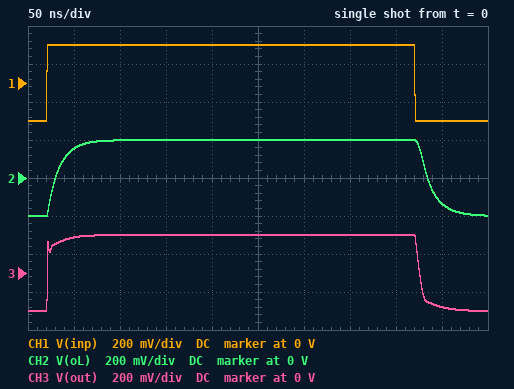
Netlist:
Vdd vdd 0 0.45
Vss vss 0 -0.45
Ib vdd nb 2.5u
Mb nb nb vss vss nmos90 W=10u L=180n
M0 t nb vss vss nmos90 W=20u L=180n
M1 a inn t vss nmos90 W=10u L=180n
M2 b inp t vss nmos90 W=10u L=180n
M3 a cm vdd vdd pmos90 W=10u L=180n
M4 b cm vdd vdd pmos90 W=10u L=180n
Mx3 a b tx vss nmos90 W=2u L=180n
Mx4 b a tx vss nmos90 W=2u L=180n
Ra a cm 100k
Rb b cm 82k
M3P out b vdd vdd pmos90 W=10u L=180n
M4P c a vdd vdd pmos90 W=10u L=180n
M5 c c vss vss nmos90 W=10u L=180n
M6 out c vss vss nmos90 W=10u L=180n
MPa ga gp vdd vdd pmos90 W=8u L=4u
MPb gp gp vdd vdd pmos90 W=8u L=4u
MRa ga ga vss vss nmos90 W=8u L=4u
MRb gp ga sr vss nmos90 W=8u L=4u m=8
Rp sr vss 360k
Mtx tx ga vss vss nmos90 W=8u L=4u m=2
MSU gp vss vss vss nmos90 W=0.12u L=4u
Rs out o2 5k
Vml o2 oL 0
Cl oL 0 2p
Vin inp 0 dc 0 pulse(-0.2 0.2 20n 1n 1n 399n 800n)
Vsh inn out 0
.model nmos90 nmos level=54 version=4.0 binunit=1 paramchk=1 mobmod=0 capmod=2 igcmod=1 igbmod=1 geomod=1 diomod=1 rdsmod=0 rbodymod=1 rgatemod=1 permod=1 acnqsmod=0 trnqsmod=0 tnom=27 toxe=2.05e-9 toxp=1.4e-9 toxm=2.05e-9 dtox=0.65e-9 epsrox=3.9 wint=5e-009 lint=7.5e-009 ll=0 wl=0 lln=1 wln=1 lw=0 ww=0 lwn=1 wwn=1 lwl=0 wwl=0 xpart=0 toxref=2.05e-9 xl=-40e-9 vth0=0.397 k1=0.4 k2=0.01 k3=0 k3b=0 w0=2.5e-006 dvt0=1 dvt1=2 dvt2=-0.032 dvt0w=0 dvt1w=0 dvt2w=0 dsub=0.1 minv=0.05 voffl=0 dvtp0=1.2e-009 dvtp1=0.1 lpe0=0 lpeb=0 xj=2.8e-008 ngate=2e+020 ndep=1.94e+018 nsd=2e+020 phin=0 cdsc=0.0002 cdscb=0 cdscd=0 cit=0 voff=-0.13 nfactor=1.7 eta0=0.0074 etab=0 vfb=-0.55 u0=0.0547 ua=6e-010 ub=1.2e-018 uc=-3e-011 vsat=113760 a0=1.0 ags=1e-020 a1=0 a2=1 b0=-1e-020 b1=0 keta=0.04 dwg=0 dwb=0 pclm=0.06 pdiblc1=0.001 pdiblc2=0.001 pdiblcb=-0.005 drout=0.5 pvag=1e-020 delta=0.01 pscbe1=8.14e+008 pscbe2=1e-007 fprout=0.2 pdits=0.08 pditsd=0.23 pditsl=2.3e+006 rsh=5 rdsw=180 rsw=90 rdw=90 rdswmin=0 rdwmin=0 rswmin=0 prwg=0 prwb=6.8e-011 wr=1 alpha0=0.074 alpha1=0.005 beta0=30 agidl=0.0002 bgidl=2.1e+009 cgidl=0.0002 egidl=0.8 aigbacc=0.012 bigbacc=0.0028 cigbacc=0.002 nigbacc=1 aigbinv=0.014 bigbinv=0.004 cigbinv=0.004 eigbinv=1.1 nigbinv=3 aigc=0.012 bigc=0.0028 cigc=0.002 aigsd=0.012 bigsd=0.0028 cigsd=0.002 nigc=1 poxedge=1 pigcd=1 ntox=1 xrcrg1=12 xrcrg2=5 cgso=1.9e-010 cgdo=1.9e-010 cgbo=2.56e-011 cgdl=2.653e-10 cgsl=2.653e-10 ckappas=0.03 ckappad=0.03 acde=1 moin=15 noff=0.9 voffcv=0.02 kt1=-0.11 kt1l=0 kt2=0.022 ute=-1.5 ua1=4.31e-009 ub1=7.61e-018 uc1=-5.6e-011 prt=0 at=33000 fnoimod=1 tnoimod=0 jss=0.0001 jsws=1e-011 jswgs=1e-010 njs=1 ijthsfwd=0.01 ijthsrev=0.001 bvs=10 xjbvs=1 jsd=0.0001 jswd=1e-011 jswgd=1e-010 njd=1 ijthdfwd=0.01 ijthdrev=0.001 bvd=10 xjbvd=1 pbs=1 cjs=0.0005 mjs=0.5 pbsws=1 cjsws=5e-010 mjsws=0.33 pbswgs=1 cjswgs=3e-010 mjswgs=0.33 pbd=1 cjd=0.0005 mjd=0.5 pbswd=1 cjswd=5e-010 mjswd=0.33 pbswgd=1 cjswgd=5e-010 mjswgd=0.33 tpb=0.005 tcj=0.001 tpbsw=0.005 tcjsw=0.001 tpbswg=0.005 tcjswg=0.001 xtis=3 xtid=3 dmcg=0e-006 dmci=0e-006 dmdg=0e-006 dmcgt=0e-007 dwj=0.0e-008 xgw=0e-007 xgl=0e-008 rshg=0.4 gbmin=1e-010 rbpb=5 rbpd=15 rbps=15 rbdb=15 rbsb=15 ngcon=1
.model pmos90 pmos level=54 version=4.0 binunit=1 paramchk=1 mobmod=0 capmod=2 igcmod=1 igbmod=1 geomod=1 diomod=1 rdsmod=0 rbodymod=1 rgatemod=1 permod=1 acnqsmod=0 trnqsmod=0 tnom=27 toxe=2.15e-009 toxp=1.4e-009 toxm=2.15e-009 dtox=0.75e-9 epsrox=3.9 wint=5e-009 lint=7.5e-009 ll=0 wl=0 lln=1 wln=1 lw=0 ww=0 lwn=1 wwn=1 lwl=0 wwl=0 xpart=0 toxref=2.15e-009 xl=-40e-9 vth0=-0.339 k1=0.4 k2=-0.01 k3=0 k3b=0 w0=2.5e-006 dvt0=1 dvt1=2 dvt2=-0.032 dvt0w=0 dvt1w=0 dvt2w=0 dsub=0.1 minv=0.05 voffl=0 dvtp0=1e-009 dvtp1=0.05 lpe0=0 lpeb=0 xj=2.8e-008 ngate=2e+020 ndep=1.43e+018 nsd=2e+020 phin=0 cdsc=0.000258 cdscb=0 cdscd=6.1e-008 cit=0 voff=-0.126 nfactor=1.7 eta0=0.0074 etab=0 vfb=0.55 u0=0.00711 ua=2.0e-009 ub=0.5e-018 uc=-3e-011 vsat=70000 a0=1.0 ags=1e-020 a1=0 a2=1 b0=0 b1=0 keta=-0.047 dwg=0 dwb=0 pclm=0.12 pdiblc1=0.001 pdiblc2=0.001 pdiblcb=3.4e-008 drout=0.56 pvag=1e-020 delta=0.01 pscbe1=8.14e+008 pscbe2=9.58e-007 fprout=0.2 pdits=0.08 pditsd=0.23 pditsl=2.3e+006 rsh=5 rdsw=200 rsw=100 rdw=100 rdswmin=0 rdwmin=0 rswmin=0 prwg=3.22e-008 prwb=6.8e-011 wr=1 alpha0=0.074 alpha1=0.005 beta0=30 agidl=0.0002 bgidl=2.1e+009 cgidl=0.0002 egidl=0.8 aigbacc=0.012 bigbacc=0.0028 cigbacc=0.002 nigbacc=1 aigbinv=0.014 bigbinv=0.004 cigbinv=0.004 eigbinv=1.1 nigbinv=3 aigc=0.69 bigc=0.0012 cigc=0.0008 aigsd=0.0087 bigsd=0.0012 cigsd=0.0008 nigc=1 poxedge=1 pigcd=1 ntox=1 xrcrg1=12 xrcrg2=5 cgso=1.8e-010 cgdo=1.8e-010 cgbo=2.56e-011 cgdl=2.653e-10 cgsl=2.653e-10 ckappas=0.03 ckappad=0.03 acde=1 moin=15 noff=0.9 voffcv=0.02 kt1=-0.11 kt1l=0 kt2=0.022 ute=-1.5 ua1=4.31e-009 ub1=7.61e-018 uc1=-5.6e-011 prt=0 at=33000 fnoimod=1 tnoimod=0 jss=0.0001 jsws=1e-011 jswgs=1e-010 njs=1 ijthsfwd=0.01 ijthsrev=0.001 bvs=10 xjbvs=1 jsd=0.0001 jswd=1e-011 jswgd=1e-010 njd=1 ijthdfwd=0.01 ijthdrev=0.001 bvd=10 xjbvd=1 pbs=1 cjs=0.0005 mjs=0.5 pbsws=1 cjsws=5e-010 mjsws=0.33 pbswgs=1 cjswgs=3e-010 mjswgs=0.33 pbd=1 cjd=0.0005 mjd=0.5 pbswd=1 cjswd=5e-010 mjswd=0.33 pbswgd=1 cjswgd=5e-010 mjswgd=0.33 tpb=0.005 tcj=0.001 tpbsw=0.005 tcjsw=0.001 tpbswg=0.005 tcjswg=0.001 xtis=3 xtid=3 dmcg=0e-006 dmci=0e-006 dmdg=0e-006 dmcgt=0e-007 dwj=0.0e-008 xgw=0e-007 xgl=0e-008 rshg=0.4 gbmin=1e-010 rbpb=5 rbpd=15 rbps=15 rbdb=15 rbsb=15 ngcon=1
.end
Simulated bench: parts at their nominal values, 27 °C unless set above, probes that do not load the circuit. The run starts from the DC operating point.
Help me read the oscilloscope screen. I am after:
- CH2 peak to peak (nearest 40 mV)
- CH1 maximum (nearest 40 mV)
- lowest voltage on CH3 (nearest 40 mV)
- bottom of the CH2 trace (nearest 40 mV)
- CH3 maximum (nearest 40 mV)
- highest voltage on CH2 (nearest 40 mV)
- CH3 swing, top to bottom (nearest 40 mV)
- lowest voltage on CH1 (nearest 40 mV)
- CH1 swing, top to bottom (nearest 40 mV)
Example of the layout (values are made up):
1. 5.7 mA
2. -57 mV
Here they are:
1. 400 mV
2. 200 mV
3. -200 mV
4. -200 mV
5. 200 mV
6. 200 mV
7. 400 mV
8. -200 mV
9. 400 mV
